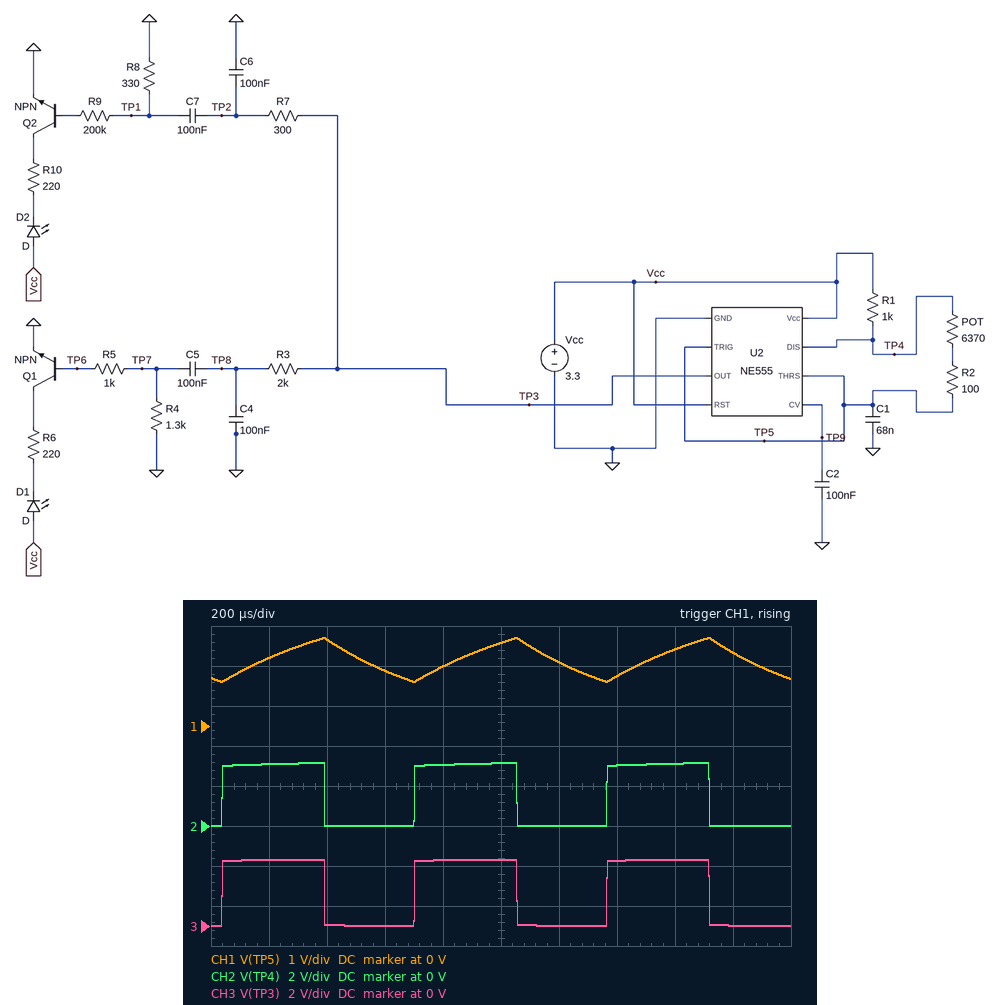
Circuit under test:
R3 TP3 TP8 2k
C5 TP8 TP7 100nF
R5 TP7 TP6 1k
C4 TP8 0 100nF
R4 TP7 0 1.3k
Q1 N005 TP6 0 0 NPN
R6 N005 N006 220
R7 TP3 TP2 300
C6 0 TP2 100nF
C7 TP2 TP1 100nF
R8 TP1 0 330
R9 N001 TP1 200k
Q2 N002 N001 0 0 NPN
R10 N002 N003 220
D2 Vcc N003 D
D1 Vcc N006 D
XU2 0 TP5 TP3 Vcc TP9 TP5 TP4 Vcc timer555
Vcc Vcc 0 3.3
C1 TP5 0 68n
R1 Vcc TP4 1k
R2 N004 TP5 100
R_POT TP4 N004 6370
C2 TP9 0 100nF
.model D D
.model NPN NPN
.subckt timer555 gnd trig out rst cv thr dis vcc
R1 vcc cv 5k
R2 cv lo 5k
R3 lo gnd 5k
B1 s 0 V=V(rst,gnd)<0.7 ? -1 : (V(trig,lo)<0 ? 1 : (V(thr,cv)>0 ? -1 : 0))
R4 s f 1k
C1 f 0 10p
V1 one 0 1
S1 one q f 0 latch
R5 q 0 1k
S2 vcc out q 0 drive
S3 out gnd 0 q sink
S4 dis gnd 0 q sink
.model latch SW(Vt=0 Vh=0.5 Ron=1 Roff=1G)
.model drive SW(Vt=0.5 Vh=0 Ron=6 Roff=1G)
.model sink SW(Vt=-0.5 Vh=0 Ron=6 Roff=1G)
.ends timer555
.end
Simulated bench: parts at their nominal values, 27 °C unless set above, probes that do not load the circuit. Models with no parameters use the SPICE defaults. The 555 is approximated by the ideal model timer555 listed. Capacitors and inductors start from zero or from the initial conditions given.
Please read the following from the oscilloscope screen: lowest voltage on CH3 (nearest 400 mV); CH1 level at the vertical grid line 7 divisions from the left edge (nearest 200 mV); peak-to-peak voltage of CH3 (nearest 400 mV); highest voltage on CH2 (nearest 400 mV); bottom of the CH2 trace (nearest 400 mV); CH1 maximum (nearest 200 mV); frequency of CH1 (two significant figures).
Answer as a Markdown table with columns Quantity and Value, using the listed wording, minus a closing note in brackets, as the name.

| Quantity | Value |
|---|---|
| lowest voltage on CH3 | 0 V |
| CH1 level at the vertical grid line 7 divisions from the left edge | 1.2 V |
| peak-to-peak voltage of CH3 | 3.2 V |
| highest voltage on CH2 | 3.2 V |
| bottom of the CH2 trace | 0 V |
| CH1 maximum | 2.2 V |
| frequency of CH1 | 1.5 kHz |
